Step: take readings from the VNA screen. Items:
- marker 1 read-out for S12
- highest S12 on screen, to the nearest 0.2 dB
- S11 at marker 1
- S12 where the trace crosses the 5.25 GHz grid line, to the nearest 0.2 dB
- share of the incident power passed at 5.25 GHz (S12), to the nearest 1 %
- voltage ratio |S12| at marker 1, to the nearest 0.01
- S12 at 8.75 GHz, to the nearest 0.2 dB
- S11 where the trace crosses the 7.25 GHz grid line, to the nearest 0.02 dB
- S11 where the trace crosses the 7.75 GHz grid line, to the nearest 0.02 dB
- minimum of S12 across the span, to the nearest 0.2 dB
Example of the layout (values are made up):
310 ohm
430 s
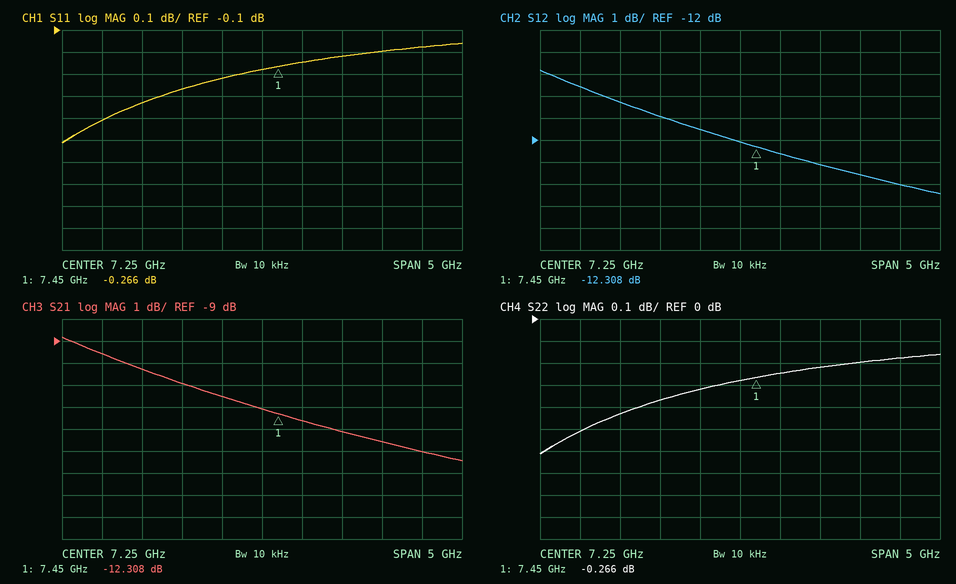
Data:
-12.308 dB
-8.8 dB
-0.266 dB
-9.6 dB
11 %
0.24
-13.6 dB
-0.28 dB
-0.24 dB
-14.4 dB
